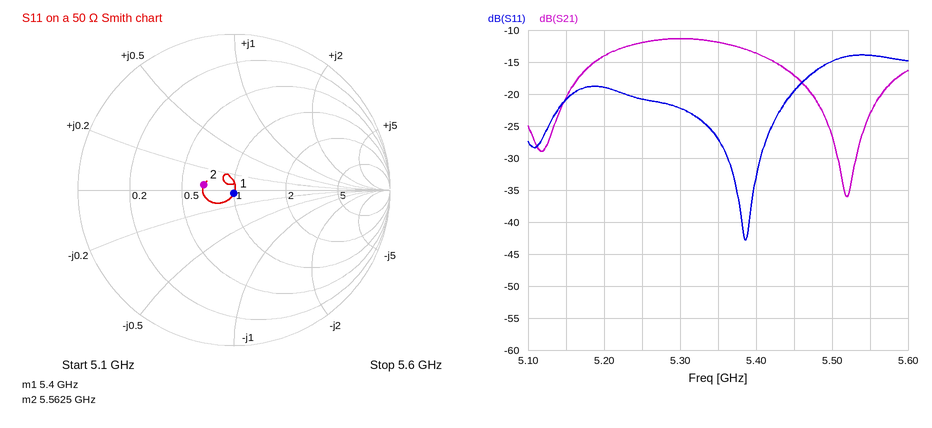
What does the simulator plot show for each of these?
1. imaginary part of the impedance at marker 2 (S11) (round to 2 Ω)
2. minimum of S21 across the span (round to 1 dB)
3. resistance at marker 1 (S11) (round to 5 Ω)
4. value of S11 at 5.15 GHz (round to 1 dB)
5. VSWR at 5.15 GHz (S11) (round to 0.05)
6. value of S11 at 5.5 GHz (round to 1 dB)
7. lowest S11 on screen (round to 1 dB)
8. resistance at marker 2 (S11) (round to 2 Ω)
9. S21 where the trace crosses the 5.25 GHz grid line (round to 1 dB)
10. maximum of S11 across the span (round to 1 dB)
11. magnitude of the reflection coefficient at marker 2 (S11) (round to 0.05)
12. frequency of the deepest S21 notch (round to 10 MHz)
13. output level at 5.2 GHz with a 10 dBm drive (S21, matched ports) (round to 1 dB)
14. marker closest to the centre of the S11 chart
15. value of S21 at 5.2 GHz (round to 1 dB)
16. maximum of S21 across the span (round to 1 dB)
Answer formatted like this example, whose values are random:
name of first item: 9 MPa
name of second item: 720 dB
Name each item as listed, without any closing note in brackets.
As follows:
imaginary part of the impedance at marker 2 (S11): +2 Ω
minimum of S21 across the span: -36 dB
resistance at marker 1 (S11): 50 Ω
value of S11 at 5.15 GHz: -21 dB
VSWR at 5.15 GHz (S11): 1.20
value of S11 at 5.5 GHz: -15 dB
lowest S11 on screen: -43 dB
resistance at marker 2 (S11): 34 Ω
S21 where the trace crosses the 5.25 GHz grid line: -12 dB
maximum of S11 across the span: -14 dB
magnitude of the reflection coefficient at marker 2 (S11): 0.20
frequency of the deepest S21 notch: 5.52 GHz
output level at 5.2 GHz with a 10 dBm drive (S21, matched ports): -4 dBm
marker closest to the centre of the S11 chart: marker 1
value of S21 at 5.2 GHz: -14 dB
maximum of S21 across the span: -11 dB
